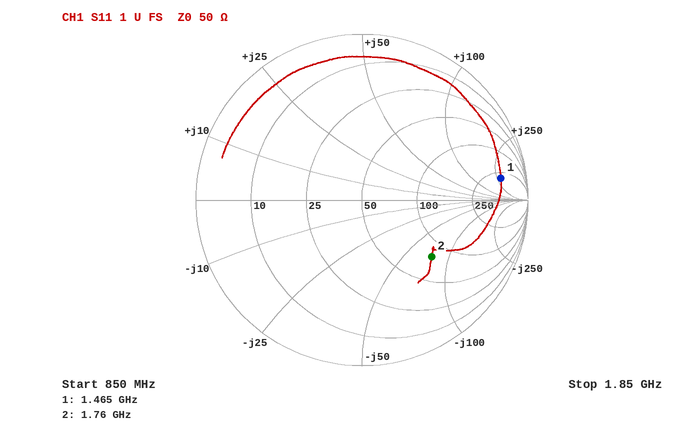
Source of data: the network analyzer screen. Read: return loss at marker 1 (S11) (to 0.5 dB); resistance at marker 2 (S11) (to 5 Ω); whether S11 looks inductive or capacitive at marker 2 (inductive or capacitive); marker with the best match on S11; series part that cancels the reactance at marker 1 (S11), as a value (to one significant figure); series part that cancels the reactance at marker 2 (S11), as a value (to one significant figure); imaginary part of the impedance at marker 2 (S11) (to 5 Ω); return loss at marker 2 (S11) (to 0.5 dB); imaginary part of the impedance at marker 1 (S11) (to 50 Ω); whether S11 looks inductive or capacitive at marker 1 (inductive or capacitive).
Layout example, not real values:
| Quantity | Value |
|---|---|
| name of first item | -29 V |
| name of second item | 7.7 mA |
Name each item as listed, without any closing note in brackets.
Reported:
| Quantity | Value |
|---|---|
| return loss at marker 1 (S11) | 1.5 dB |
| resistance at marker 2 (S11) | 80 Ω |
| whether S11 looks inductive or capacitive at marker 2 | capacitive |
| marker with the best match on S11 | marker 2 |
| series part that cancels the reactance at marker 1 (S11), as a value | 400 fF |
| series part that cancels the reactance at marker 2 (S11), as a value | 7 nH |
| imaginary part of the impedance at marker 2 (S11) | -75 Ω |
| return loss at marker 2 (S11) | 5.5 dB |
| imaginary part of the impedance at marker 1 (S11) | +300 Ω |
| whether S11 looks inductive or capacitive at marker 1 | inductive |
